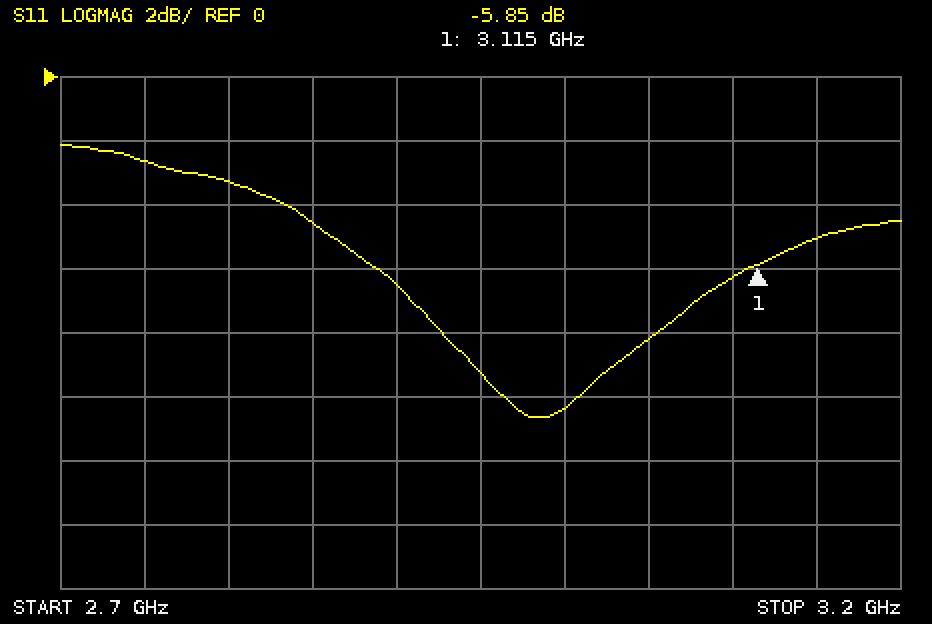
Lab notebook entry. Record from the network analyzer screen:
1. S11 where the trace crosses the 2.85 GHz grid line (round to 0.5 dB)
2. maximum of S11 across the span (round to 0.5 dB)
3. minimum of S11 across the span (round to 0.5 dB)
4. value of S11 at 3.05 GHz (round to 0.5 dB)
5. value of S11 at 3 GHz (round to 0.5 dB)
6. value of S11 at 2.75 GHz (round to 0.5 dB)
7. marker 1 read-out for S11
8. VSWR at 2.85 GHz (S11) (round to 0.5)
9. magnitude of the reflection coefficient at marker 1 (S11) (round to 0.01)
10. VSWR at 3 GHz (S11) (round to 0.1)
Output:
-4.5 dB
-2.0 dB
-10.5 dB
-8.0 dB
-10.5 dB
-2.5 dB
-5.85 dB
4.0
0.51
1.9
